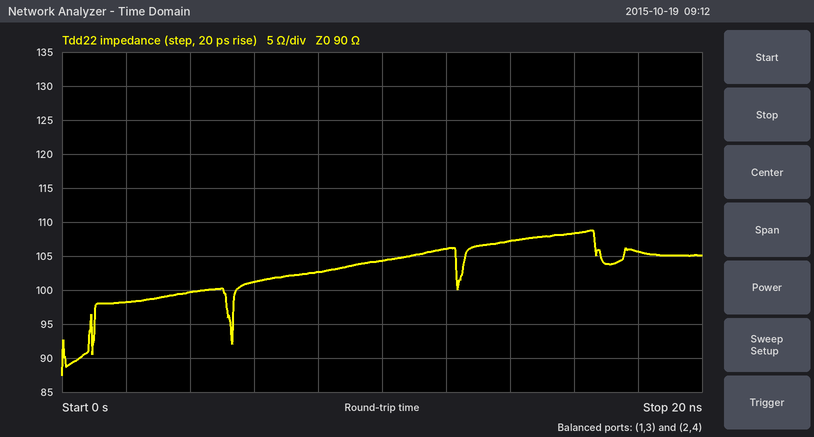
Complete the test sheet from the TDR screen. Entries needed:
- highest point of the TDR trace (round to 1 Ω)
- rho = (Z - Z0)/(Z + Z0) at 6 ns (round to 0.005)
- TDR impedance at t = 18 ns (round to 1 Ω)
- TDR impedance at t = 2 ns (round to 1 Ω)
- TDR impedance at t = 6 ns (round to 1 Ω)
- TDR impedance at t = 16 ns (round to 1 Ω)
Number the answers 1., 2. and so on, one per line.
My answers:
1. 109 Ω
2. +0.060
3. 106 Ω
4. 98 Ω
5. 101 Ω
6. 108 Ω
